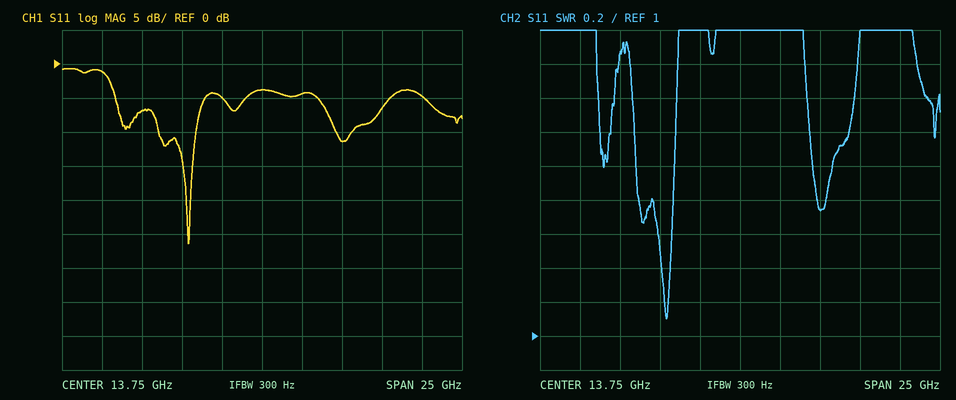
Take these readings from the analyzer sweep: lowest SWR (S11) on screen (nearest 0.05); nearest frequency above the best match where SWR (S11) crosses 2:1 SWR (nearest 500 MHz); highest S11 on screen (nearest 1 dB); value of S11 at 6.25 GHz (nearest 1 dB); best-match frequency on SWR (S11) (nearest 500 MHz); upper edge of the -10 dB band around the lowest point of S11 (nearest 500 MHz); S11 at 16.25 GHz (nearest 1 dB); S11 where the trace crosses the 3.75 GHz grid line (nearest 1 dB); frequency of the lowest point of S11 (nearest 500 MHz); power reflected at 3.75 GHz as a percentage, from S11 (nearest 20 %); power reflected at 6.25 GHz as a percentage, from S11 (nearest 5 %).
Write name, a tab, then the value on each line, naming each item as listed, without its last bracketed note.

lowest SWR (S11) on screen	1.10
nearest frequency above the best match where SWR (S11) crosses 2:1 SWR	9.5 GHz
highest S11 on screen	-1 dB
value of S11 at 6.25 GHz	-7 dB
best-match frequency on SWR (S11)	9.0 GHz
upper edge of the -10 dB band around the lowest point of S11	9.5 GHz
S11 at 16.25 GHz	-4 dB
S11 where the trace crosses the 3.75 GHz grid line	-1 dB
frequency of the lowest point of S11	9.0 GHz
power reflected at 3.75 GHz as a percentage, from S11	80 %
power reflected at 6.25 GHz as a percentage, from S11	20 %
